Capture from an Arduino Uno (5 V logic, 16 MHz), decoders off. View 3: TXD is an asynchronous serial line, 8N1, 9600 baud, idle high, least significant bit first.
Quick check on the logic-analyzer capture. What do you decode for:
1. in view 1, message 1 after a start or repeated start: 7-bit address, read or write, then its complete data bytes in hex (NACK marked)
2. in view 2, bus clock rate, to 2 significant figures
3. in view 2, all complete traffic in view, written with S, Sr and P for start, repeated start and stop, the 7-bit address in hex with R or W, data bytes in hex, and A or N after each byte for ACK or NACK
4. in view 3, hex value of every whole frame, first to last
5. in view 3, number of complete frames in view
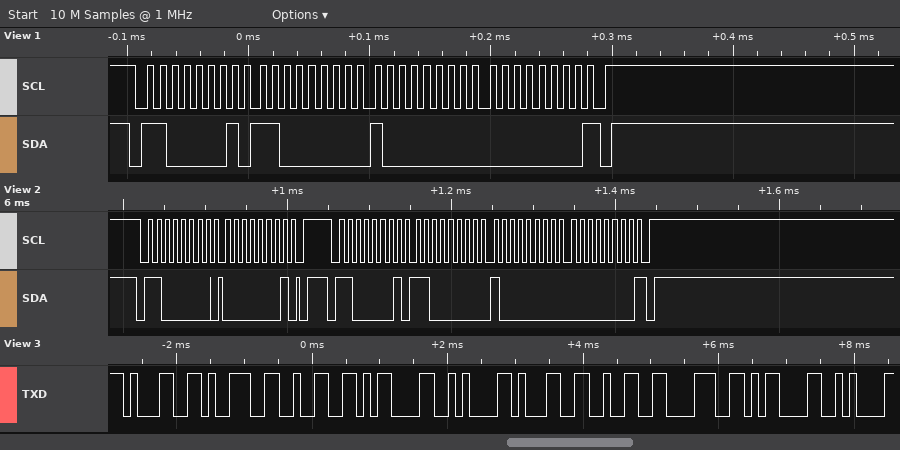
0x60 read: C0 80 00 NACK
100 kHz
S 60W A 01 A P S 60R A C0 A 80 A 00 N P
31 39 32 0D 0A 31 32 38 0D 0A
10
